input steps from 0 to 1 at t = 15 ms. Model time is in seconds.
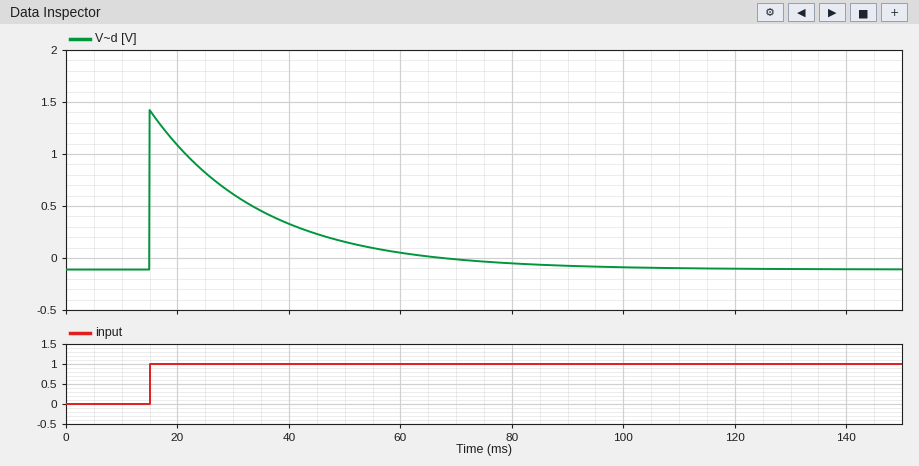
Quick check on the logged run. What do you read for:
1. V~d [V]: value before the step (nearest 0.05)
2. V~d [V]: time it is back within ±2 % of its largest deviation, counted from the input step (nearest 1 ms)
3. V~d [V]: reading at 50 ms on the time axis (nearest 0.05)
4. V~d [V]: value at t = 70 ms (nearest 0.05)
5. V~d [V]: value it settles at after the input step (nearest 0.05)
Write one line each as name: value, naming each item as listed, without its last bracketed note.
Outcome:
V~d [V]: value before the step: -0.10
V~d [V]: time it is back within ±2 % of its largest deviation, counted from the input step: 78 ms
V~d [V]: reading at 50 ms on the time axis: 0.15
V~d [V]: value at t = 70 ms: 0.00
V~d [V]: value it settles at after the input step: -0.10
